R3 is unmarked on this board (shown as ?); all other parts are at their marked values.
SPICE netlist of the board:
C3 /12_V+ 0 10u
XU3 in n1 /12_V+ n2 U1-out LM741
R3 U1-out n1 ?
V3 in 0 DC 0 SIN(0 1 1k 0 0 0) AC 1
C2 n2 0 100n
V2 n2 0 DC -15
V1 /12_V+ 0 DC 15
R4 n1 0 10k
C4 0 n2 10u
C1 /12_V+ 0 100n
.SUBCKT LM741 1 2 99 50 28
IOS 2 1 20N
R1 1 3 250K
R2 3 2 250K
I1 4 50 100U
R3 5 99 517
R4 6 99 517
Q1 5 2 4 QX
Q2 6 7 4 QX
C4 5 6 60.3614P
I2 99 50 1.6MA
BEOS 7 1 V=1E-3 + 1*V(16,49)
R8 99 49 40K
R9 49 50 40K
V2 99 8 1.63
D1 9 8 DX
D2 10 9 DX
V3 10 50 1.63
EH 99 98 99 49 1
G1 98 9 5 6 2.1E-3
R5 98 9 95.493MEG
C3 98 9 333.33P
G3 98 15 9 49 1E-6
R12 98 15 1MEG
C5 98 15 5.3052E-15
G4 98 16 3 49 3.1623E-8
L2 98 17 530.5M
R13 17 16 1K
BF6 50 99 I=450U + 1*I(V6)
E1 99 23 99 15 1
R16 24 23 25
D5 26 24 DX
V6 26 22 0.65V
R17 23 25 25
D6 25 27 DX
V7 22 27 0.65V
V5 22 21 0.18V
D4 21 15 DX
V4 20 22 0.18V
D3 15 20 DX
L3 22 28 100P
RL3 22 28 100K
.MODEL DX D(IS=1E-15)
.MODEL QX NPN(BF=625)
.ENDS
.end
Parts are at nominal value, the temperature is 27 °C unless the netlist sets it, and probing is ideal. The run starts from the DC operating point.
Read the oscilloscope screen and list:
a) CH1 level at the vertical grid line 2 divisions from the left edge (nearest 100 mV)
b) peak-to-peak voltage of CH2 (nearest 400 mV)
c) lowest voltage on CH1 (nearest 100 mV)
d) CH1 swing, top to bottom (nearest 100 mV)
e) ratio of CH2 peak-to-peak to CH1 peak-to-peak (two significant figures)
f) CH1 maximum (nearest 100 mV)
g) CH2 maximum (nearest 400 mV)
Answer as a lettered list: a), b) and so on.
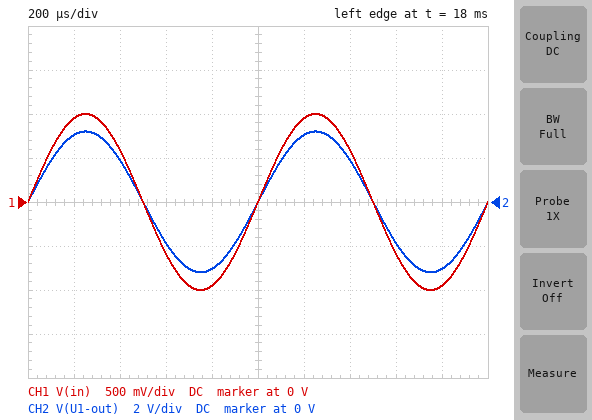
a) 600 mV
b) 6.4 V
c) -1.0 V
d) 2.0 V
e) 3.2
f) 1.0 V
g) 3.2 V
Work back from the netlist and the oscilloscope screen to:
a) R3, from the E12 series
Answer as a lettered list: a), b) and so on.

a) 22 kΩ
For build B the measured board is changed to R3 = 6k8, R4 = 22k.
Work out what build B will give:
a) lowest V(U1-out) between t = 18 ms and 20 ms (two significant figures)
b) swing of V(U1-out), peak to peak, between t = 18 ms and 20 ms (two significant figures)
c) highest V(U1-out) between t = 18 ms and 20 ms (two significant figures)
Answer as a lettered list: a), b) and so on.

a) -1.3 V
b) 2.6 V
c) 1.3 V
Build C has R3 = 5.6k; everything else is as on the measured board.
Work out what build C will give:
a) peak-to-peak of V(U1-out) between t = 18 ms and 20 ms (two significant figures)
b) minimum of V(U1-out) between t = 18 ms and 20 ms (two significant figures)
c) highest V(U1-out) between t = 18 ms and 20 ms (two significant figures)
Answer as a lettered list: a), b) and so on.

a) 3.1 V
b) -1.6 V
c) 1.6 V
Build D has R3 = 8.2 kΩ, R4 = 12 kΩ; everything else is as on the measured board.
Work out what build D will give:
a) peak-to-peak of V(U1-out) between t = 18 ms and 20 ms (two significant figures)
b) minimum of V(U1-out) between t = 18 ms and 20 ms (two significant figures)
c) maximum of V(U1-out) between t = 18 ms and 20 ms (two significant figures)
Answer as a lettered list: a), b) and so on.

a) 3.4 V
b) -1.7 V
c) 1.7 V
